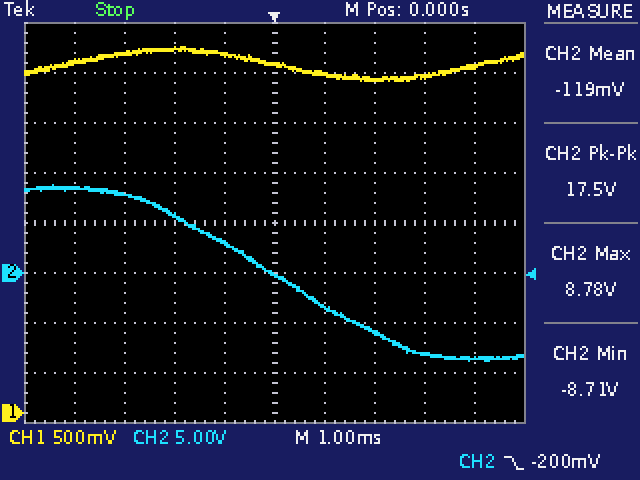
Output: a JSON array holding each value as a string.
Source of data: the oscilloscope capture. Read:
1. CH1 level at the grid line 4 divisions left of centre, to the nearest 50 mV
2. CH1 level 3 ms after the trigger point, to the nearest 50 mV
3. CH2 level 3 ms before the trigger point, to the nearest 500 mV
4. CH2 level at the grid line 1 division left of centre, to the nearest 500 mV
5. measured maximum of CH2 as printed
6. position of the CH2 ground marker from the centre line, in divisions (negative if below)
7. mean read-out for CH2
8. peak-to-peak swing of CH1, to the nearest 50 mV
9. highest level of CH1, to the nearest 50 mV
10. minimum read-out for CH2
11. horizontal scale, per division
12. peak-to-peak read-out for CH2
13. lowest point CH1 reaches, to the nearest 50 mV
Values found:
["3.50 V", "3.35 V", "8.0 V", "3.0 V", "8.78 V", "-1.0 div", "-119 mV", "350 mV", "3.65 V", "-8.71 V", "1 ms", "17.5 V", "3.30 V"]
